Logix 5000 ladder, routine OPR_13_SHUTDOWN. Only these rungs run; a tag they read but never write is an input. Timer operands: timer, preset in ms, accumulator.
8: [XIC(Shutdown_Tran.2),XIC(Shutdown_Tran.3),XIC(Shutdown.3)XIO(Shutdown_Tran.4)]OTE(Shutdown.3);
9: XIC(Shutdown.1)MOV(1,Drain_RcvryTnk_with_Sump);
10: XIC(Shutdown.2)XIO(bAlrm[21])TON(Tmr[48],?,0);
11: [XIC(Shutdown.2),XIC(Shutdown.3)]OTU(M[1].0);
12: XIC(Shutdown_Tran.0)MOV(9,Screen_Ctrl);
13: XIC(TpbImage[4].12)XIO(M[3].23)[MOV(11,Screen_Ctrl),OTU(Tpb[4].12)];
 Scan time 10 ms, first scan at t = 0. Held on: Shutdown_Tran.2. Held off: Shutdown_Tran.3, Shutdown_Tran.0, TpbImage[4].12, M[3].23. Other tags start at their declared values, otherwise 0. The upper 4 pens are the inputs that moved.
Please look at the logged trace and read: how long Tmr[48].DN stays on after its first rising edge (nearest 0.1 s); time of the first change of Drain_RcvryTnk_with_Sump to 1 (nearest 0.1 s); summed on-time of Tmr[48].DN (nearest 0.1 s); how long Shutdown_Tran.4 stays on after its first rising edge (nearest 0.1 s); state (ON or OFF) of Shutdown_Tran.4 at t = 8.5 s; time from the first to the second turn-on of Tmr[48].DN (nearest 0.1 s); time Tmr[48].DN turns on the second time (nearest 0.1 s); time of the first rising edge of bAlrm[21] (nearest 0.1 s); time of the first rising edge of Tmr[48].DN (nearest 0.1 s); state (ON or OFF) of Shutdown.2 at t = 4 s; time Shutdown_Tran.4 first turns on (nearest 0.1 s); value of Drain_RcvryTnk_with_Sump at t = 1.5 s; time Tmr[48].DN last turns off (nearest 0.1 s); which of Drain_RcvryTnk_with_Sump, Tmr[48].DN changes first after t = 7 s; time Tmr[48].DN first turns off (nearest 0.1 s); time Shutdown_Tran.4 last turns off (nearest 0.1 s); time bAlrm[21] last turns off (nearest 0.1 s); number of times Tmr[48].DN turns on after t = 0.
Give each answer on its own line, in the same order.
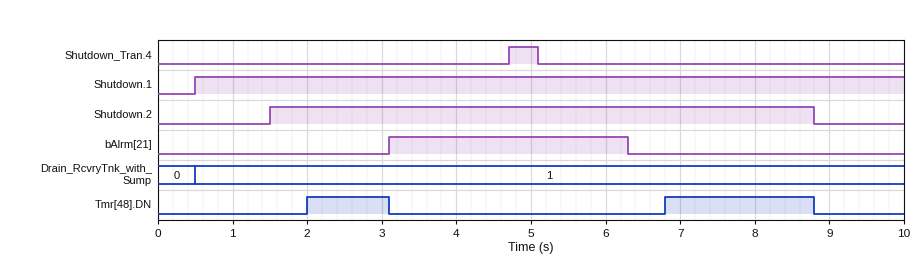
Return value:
1.1 s
0.5 s
3.1 s
0.4 s
OFF
4.8 s
6.8 s
3.1 s
2.0 s
ON
4.7 s
1
8.8 s
Tmr[48].DN
3.1 s
5.1 s
6.3 s
2
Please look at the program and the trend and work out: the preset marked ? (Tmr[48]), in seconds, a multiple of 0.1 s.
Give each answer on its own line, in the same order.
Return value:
0.5 s
